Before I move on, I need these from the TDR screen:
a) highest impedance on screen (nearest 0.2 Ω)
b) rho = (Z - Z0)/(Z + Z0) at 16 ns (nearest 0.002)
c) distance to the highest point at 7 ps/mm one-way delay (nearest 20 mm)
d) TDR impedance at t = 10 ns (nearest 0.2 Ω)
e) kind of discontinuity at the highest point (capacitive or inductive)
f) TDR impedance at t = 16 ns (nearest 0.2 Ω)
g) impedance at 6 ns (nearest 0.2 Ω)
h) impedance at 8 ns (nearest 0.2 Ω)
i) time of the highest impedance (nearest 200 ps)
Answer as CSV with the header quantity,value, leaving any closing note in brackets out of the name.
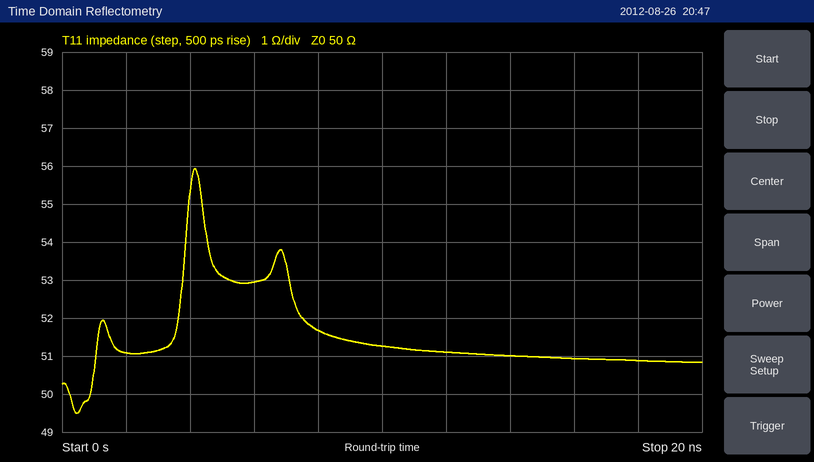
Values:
quantity,value
highest impedance on screen,56.0 Ω
rho = (Z - Z0)/(Z + Z0) at 16 ns,+0.010
distance to the highest point at 7 ps/mm one-way delay,300 mm
TDR impedance at t = 10 ns,51.2 Ω
kind of discontinuity at the highest point,inductive
TDR impedance at t = 16 ns,51.0 Ω
impedance at 6 ns,53.0 Ω
impedance at 8 ns,51.6 Ω
time of the highest impedance,4.2 ns
